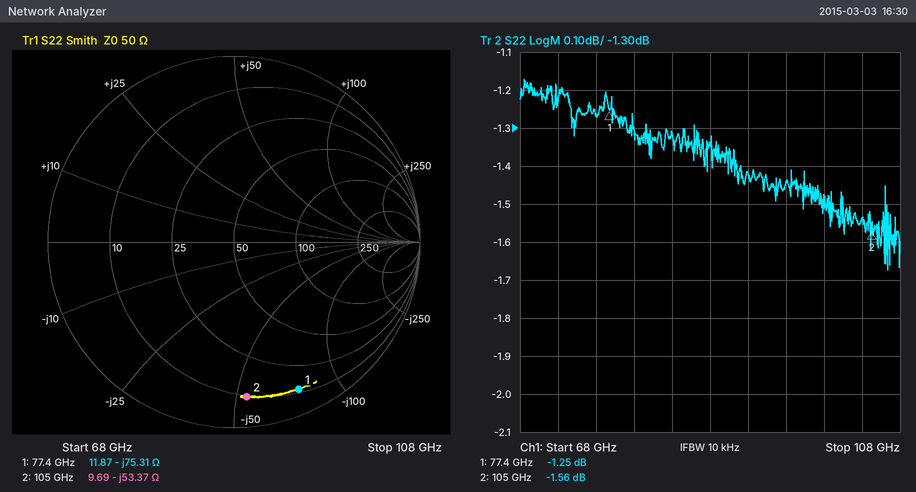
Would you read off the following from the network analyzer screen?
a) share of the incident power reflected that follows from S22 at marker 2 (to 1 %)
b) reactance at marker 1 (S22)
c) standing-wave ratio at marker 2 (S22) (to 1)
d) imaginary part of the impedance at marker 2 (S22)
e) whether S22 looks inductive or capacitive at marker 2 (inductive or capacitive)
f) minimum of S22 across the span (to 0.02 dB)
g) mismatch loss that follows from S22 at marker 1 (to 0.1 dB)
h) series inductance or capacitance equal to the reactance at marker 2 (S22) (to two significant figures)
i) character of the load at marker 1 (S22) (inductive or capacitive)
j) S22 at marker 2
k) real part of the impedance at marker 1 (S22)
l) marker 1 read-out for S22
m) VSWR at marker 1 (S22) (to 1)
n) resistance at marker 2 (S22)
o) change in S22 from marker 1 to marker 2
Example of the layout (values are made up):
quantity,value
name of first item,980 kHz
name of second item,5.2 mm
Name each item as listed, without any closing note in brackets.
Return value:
quantity,value
share of the incident power reflected that follows from S22 at marker 2,70 %
reactance at marker 1,-75.31 Ω
standing-wave ratio at marker 2 (S22),11
imaginary part of the impedance at marker 2,-53.37 Ω
whether S22 looks inductive or capacitive at marker 2,capacitive
minimum of S22 across the span,-1.68 dB
mismatch loss that follows from S22 at marker 1,6.0 dB
series inductance or capacitance equal to the reactance at marker 2 (S22),28 fF
character of the load at marker 1 (S22),capacitive
S22 at marker 2,-1.56 dB
real part of the impedance at marker 1,11.87 Ω
marker 1 read-out for S22,-1.25 dB
VSWR at marker 1 (S22),14
resistance at marker 2,9.69 Ω
change in S22 from marker 1 to marker 2,-0.31 dB
